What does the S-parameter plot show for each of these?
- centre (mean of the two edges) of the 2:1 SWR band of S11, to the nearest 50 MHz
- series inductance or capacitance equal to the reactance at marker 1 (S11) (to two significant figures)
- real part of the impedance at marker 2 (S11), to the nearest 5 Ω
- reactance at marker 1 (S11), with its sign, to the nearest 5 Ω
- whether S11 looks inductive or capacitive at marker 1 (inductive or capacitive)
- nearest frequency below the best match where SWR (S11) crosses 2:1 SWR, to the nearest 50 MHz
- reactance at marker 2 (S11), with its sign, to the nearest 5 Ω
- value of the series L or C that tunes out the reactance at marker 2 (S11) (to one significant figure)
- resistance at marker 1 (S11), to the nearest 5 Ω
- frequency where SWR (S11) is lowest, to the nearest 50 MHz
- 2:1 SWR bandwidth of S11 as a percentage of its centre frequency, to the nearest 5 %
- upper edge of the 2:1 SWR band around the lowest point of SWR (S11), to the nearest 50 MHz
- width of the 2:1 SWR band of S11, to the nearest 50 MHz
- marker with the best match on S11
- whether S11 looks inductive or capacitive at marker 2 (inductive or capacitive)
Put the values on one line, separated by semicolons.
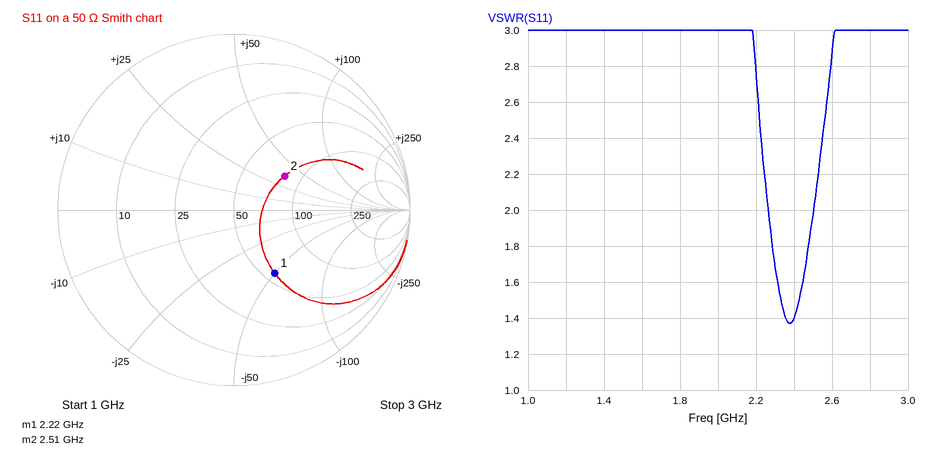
2.40 GHz; 1.4 pF; 80 Ω; -50 Ω; capacitive; 2.25 GHz; +35 Ω; 2 pF; 55 Ω; 2.40 GHz; 10 %; 2.50 GHz; 250 MHz; marker 2; inductive
